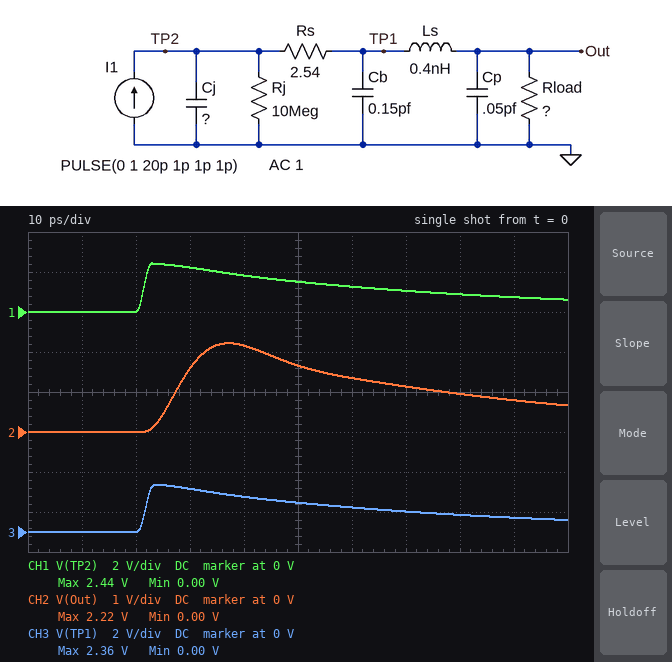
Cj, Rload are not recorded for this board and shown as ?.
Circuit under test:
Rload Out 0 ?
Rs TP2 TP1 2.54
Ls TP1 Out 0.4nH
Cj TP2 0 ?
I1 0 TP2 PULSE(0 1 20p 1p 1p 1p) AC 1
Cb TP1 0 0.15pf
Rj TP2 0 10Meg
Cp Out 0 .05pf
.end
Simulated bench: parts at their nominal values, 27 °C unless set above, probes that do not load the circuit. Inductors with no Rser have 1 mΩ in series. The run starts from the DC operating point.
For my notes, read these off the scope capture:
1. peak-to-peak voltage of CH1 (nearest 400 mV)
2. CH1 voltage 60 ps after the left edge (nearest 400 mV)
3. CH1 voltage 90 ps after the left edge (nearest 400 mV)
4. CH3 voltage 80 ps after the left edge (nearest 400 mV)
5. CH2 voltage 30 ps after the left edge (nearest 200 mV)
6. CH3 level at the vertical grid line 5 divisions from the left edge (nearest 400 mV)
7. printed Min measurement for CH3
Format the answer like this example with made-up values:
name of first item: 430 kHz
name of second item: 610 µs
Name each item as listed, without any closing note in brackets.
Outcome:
peak-to-peak voltage of CH1: 2.4 V
CH1 voltage 60 ps after the left edge: 1.2 V
CH1 voltage 90 ps after the left edge: 800 mV
CH3 voltage 80 ps after the left edge: 800 mV
CH2 voltage 30 ps after the left edge: 1.6 V
CH3 level at the vertical grid line 5 divisions from the left edge: 1.6 V
printed Min measurement for CH3: 0.00 V
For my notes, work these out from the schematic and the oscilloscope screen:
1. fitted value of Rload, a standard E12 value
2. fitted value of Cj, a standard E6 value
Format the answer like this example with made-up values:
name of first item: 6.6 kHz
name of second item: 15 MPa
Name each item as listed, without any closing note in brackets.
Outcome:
fitted value of Rload, a standard E12 value: 68 Ω
fitted value of Cj, a standard E6 value: 680 fF
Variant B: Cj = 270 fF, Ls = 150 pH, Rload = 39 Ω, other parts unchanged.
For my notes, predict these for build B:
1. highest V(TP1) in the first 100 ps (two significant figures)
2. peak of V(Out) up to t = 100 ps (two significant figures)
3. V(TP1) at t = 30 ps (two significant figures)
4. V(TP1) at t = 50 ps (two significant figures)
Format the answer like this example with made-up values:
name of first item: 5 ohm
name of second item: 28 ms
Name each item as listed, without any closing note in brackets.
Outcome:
highest V(TP1) in the first 100 ps: 4.6 V
peak of V(Out) up to t = 100 ps: 3.9 V
V(TP1) at t = 30 ps: 3.1 V
V(TP1) at t = 50 ps: 780 mV
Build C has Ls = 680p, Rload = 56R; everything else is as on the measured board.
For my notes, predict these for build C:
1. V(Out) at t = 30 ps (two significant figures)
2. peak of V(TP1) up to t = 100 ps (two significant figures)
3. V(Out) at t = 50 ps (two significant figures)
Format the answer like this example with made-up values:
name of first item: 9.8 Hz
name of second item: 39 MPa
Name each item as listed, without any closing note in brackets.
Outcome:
V(Out) at t = 30 ps: 940 mV
peak of V(TP1) up to t = 100 ps: 2.4 V
V(Out) at t = 50 ps: 1.8 V
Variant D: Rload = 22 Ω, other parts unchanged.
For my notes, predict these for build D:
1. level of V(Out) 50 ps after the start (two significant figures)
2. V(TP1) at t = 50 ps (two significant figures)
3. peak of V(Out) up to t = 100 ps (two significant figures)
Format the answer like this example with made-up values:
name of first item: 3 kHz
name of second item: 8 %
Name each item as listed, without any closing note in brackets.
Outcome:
level of V(Out) 50 ps after the start: 1.2 V
V(TP1) at t = 50 ps: 790 mV
peak of V(Out) up to t = 100 ps: 1.3 V
